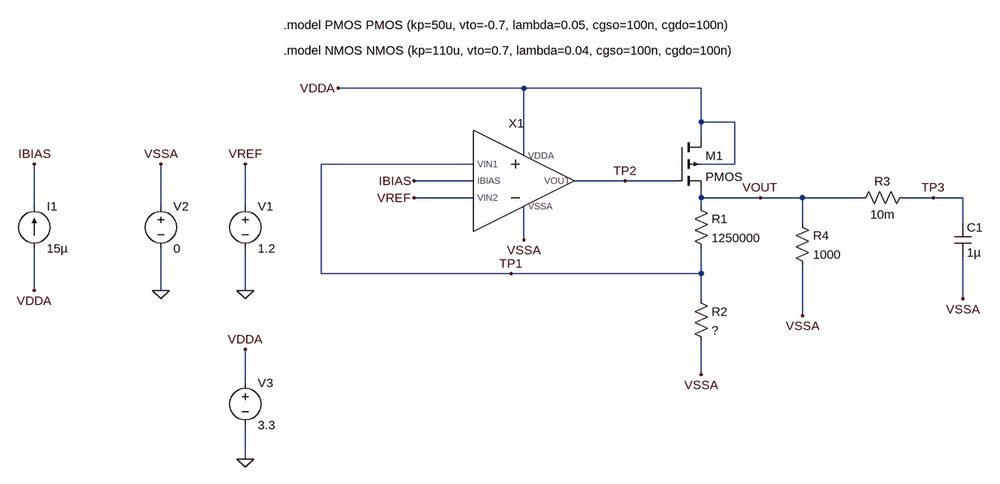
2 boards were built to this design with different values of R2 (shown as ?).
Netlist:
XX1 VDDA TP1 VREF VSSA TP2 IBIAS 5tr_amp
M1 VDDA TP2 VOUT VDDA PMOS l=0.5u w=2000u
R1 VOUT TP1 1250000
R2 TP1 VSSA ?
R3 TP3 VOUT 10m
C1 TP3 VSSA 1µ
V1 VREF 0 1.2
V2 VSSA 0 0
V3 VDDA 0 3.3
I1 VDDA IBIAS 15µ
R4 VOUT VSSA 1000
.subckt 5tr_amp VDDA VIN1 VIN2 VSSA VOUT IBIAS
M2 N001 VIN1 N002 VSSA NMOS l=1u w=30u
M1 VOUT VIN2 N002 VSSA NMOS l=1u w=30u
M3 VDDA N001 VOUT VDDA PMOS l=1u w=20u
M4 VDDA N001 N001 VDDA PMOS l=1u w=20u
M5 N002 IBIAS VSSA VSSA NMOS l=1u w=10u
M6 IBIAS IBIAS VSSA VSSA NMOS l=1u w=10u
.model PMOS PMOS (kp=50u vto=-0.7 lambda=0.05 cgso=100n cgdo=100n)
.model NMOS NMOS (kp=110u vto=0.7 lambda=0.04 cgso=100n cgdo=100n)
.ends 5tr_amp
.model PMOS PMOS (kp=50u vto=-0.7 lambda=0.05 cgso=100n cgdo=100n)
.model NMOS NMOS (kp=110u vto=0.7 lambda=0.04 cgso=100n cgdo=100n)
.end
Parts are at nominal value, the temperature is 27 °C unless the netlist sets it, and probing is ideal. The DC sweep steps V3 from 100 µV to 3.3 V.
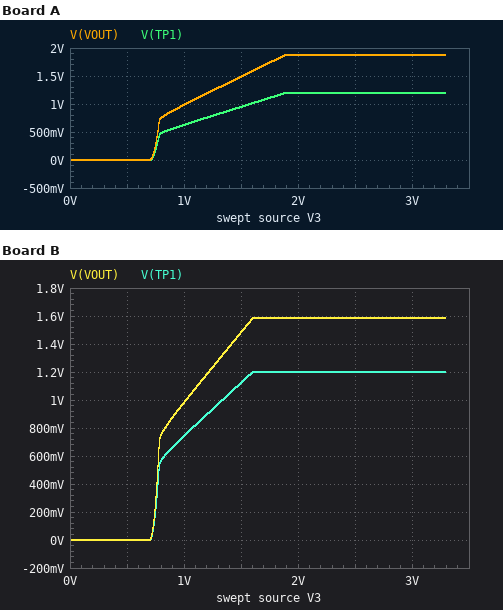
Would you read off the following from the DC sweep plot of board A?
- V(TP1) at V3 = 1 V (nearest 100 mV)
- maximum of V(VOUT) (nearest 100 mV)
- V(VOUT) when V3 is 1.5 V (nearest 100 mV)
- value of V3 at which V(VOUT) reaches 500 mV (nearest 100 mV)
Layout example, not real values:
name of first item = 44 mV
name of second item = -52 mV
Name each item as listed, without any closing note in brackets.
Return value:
V(TP1) at V3 = 1 V = 600 mV
maximum of V(VOUT) = 1.9 V
V(VOUT) when V3 is 1.5 V = 1.5 V
value of V3 at which V(VOUT) reaches 500 mV = 800 mV
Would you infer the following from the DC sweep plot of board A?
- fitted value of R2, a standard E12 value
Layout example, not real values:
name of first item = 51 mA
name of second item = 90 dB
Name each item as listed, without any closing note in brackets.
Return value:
fitted value of R2, a standard E12 value = 2.2 MΩ
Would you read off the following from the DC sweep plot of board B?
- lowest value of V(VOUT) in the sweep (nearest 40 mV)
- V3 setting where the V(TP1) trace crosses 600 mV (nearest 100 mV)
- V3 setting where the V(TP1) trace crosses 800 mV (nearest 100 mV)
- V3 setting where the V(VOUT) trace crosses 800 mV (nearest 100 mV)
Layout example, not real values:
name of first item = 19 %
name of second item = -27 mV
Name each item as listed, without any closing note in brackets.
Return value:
lowest value of V(VOUT) in the sweep = 0 V
V3 setting where the V(TP1) trace crosses 600 mV = 800 mV
V3 setting where the V(TP1) trace crosses 800 mV = 1.1 V
V3 setting where the V(VOUT) trace crosses 800 mV = 800 mV
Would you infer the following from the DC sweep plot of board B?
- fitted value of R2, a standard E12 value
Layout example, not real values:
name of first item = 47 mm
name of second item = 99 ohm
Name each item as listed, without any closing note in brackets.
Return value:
fitted value of R2, a standard E12 value = 3.9 MΩ
